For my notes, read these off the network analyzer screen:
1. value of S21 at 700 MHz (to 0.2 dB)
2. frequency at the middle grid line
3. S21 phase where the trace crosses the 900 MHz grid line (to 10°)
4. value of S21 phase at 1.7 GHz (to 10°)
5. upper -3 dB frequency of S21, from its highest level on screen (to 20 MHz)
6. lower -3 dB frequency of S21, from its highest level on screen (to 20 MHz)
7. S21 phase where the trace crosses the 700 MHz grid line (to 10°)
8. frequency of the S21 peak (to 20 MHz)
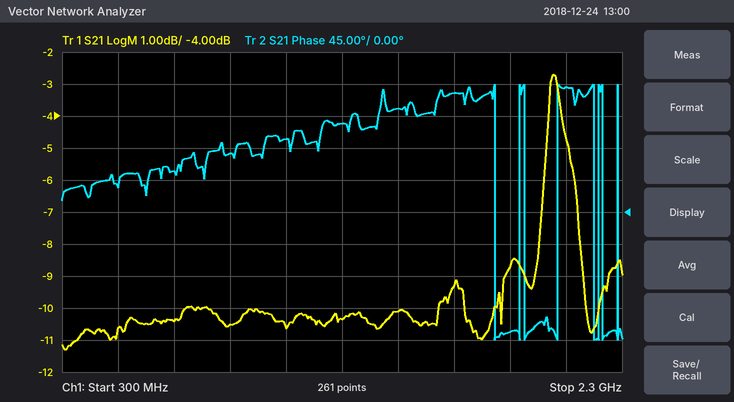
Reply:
-10.4 dB
1.3 GHz
80°
170°
2.12 GHz
2.02 GHz
60°
2.06 GHz
